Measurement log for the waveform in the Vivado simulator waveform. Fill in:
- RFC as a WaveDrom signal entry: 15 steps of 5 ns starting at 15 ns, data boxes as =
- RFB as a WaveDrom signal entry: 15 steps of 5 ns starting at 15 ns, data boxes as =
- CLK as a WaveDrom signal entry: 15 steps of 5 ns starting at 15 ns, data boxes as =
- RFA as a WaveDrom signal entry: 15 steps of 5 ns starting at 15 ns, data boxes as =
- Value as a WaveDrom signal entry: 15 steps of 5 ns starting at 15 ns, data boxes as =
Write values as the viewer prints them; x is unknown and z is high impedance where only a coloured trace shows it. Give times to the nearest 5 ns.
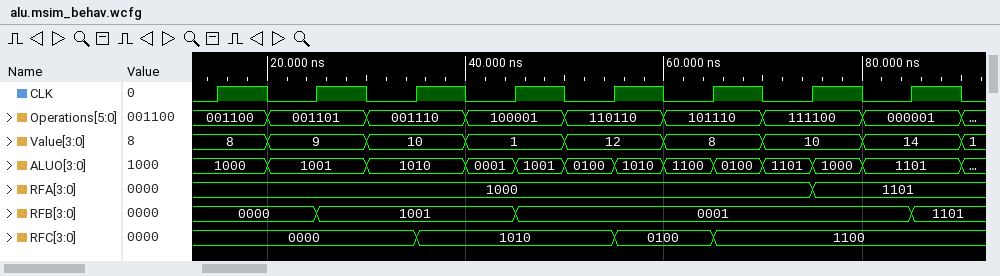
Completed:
{name: 'RFC', wave: '=...=...=.=....', data: '0000 1010 0100 1100'}
{name: 'RFB', wave: '=.=...=.......=', data: '0000 1001 0001 1101'}
{name: 'CLK', wave: '101010101010101'}
{name: 'RFA', wave: '=...........=..', data: '1000 1101'}
{name: 'Value', wave: '==.=.=.=.=.=.=.', data: '8 9 10 1 12 8 10 14'}
